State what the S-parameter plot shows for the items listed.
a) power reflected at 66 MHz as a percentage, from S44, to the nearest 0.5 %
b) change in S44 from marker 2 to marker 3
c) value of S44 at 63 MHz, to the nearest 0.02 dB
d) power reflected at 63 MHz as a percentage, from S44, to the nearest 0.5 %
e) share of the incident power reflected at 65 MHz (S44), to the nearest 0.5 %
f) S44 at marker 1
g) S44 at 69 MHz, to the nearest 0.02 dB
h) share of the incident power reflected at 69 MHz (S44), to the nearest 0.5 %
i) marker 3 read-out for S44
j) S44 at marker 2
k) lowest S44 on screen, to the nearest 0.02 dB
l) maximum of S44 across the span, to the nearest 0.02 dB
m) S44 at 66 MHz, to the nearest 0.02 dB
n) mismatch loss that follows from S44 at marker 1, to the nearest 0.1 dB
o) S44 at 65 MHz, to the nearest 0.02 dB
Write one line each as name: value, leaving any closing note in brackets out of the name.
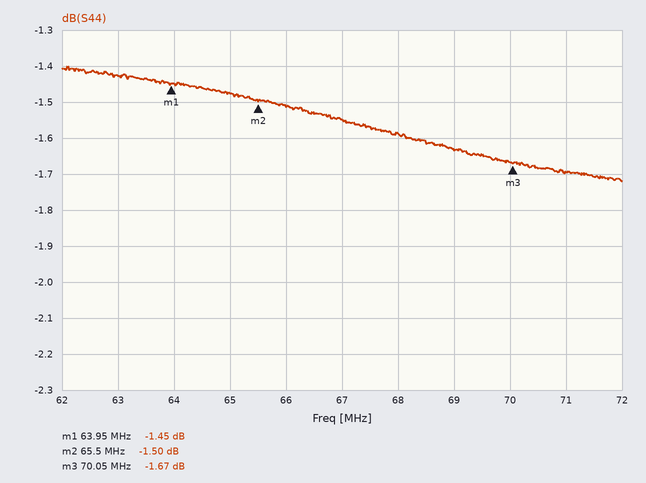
power reflected at 66 MHz as a percentage, from S44, to the nearest 0.5 %: 70.5 %
change in S44 from marker 2 to marker 3: -0.17 dB
value of S44 at 63 MHz, to the nearest 0.02 dB: -1.42 dB
power reflected at 63 MHz as a percentage, from S44, to the nearest 0.5 %: 72.0 %
share of the incident power reflected at 65 MHz (S44), to the nearest 0.5 %: 71.0 %
S44 at marker 1: -1.45 dB
S44 at 69 MHz, to the nearest 0.02 dB: -1.64 dB
share of the incident power reflected at 69 MHz (S44), to the nearest 0.5 %: 68.5 %
marker 3 read-out for S44: -1.67 dB
S44 at marker 2: -1.50 dB
lowest S44 on screen, to the nearest 0.02 dB: -1.72 dB
maximum of S44 across the span, to the nearest 0.02 dB: -1.40 dB
S44 at 66 MHz, to the nearest 0.02 dB: -1.52 dB
mismatch loss that follows from S44 at marker 1, to the nearest 0.1 dB: 5.5 dB
S44 at 65 MHz, to the nearest 0.02 dB: -1.48 dB
